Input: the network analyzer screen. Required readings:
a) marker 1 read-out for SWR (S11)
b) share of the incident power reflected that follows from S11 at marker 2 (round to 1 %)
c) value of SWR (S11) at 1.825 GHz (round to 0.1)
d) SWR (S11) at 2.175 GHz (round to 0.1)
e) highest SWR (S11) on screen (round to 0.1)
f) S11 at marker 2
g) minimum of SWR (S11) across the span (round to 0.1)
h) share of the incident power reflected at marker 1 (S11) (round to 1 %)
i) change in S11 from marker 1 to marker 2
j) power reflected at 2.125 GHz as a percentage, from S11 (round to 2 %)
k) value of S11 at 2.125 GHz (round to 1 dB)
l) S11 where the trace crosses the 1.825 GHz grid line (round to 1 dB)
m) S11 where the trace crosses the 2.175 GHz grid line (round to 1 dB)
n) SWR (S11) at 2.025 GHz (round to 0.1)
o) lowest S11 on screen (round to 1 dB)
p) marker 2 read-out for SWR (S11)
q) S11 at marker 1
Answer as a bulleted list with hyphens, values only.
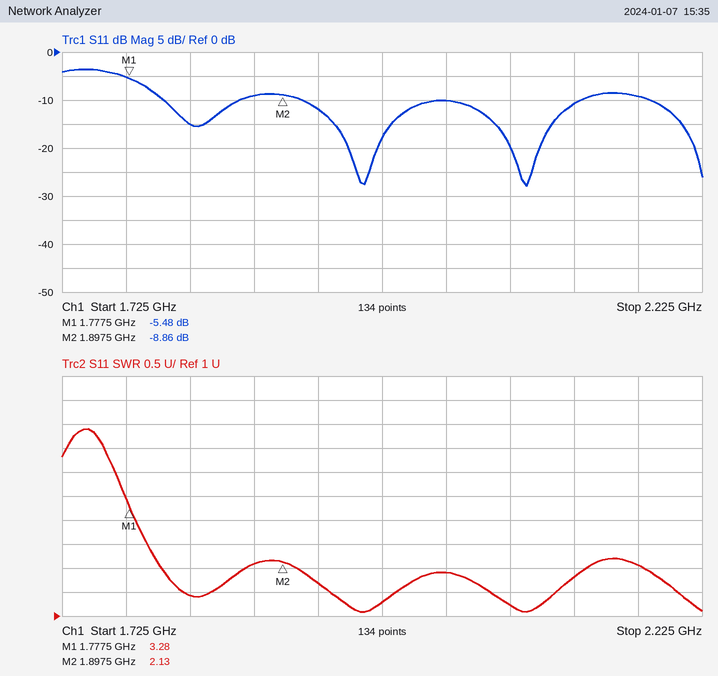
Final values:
- 3.28
- 13 %
- 1.4
- 2.1
- 4.9
- -8.86 dB
- 1.1
- 28 %
- -3.38 dB
- 8 %
- -11 dB
- -15 dB
- -9 dB
- 1.9
- -28 dB
- 2.13
- -5.48 dB
